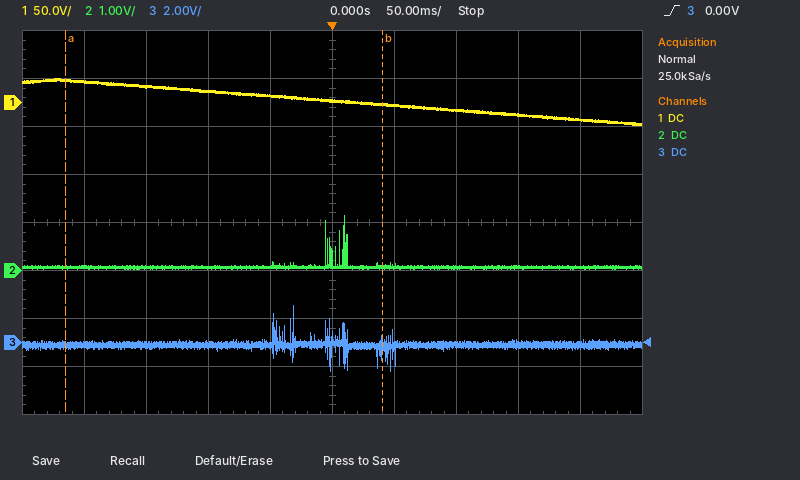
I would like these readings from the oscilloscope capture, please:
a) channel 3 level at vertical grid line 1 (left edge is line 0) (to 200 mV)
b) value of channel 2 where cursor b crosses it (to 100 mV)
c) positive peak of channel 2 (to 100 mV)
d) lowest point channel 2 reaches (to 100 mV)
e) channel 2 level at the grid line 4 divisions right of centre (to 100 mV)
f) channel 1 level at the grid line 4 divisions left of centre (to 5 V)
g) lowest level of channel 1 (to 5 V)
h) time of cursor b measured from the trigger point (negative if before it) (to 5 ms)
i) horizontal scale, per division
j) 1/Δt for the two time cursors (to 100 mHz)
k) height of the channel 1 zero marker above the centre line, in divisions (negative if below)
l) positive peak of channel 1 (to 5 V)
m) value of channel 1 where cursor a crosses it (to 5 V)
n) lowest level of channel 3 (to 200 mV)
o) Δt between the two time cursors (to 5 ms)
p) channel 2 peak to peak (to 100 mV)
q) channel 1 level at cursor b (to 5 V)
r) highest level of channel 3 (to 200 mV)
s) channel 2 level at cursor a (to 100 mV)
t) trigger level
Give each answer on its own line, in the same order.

0.0 V
100 mV
1.1 V
0.0 V
100 mV
20 V
-25 V
+40 ms
50 ms
3.9 Hz
+2.5 div
25 V
25 V
-1.2 V
255 ms
1.1 V
0 V
1.6 V
100 mV
0.00 V
